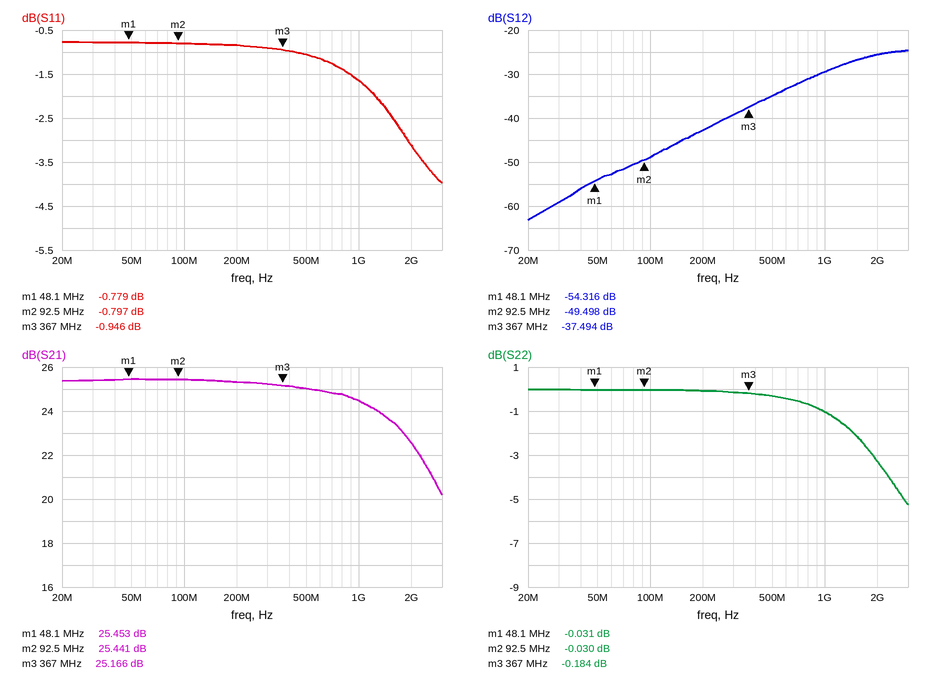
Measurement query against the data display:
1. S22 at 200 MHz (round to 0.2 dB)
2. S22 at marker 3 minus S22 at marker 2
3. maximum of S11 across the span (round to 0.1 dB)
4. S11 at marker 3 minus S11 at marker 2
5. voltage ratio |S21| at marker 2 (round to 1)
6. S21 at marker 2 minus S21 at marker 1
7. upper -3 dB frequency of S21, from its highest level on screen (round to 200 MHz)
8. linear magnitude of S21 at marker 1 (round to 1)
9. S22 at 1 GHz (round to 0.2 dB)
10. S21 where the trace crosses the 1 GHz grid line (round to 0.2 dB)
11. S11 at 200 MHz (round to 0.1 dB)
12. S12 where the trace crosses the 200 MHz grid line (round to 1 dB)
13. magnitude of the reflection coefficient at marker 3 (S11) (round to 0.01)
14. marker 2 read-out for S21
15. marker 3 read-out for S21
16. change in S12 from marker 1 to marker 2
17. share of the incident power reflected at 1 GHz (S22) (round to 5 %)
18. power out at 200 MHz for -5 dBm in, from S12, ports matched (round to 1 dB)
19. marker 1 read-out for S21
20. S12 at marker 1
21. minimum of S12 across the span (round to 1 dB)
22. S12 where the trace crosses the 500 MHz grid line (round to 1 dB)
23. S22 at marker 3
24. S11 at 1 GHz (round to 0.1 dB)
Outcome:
0.0 dB
-0.154 dB
-0.8 dB
-0.149 dB
19
-0.012 dB
2.0 GHz
19
-1.0 dB
24.4 dB
-0.8 dB
-43 dB
0.90
25.441 dB
25.166 dB
4.818 dB
80 %
-48 dBm
25.453 dB
-54.316 dB
-63 dB
-35 dB
-0.184 dB
-1.6 dB
